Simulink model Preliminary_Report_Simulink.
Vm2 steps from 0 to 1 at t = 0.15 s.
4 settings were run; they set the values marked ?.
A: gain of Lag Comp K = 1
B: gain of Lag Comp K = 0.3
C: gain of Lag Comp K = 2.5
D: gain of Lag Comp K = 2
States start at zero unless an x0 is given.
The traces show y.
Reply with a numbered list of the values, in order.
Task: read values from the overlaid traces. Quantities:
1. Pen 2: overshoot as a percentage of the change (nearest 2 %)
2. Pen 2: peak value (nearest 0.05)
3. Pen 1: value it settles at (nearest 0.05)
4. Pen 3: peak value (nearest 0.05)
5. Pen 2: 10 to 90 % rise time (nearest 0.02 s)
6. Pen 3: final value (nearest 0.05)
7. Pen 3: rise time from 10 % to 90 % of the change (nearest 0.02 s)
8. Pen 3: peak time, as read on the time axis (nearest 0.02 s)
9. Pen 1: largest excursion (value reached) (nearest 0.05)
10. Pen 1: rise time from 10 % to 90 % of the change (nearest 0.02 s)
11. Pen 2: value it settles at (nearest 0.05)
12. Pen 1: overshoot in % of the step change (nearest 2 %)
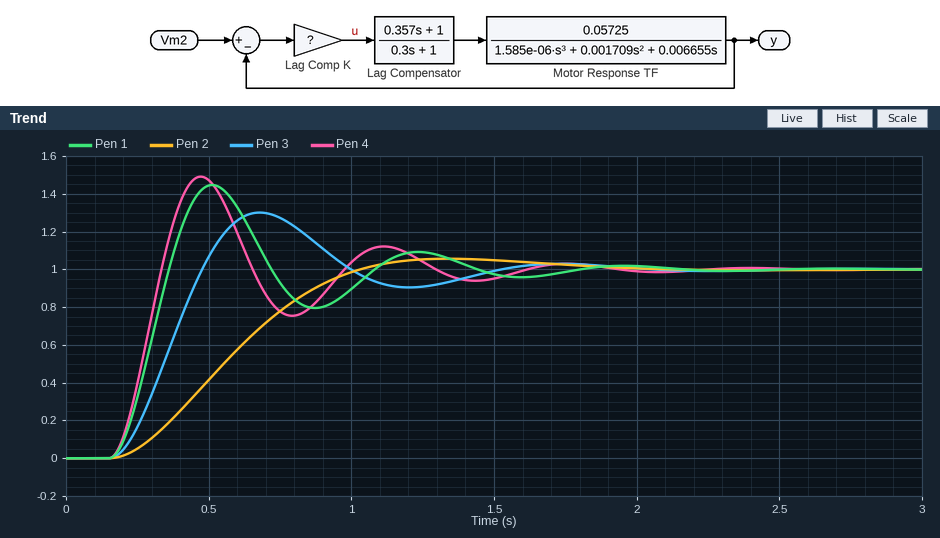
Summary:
1. 6 %
2. 1.05
3. 1.00
4. 1.30
5. 0.58 s
6. 1.00
7. 0.22 s
8. 0.68 s
9. 1.45
10. 0.14 s
11. 1.00
12. 44 %
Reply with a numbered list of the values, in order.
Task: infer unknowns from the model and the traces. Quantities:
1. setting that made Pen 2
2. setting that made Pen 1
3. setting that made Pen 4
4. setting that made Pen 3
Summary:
1. B
2. D
3. C
4. A
